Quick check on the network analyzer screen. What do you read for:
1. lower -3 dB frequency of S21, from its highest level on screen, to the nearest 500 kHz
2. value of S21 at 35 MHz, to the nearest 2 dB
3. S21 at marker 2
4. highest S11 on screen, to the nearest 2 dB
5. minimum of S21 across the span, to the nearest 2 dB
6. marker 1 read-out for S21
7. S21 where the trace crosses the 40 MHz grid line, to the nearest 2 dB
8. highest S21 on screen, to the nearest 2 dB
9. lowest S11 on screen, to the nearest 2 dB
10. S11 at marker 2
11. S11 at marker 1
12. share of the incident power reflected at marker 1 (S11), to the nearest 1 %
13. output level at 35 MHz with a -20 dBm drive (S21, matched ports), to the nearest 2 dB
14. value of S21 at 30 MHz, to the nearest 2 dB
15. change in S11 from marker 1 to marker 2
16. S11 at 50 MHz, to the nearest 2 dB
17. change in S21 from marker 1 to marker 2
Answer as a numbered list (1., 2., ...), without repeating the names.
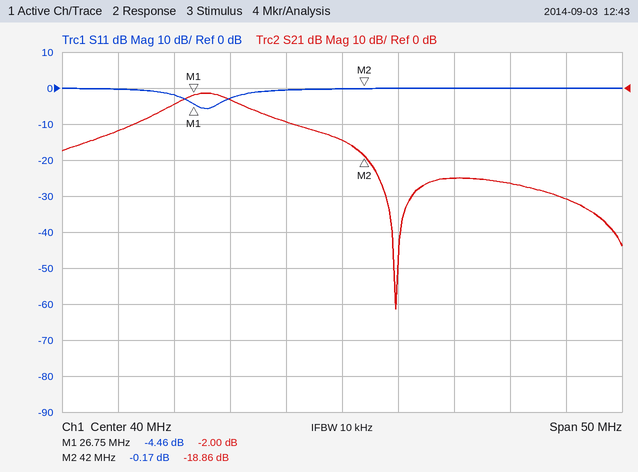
1. 25.0 MHz
2. -10 dB
3. -18.86 dB
4. 0 dB
5. -62 dB
6. -2.00 dB
7. -14 dB
8. -2 dB
9. -6 dB
10. -0.17 dB
11. -4.46 dB
12. 36 %
13. -30 dBm
14. -4 dB
15. 4.29 dB
16. 0 dB
17. -16.86 dB
